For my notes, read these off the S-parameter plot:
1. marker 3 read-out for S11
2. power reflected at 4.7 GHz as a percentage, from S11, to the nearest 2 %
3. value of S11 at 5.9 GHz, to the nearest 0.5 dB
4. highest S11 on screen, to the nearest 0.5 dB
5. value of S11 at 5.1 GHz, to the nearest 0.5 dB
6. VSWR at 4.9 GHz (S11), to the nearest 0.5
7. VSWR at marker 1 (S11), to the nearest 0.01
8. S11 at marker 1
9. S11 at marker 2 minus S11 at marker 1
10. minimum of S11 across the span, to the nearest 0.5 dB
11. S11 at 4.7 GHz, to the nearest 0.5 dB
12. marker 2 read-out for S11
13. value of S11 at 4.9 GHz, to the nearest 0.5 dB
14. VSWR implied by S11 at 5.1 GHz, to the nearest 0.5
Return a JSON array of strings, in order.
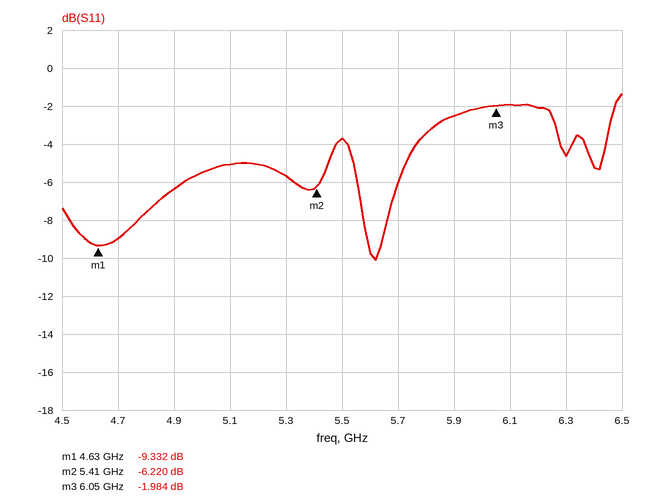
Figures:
["-1.984 dB", "12 %", "-2.5 dB", "-1.5 dB", "-5.0 dB", "3.0", "2.04", "-9.332 dB", "3.112 dB", "-10.0 dB", "-9.0 dB", "-6.220 dB", "-6.5 dB", "3.5"]
